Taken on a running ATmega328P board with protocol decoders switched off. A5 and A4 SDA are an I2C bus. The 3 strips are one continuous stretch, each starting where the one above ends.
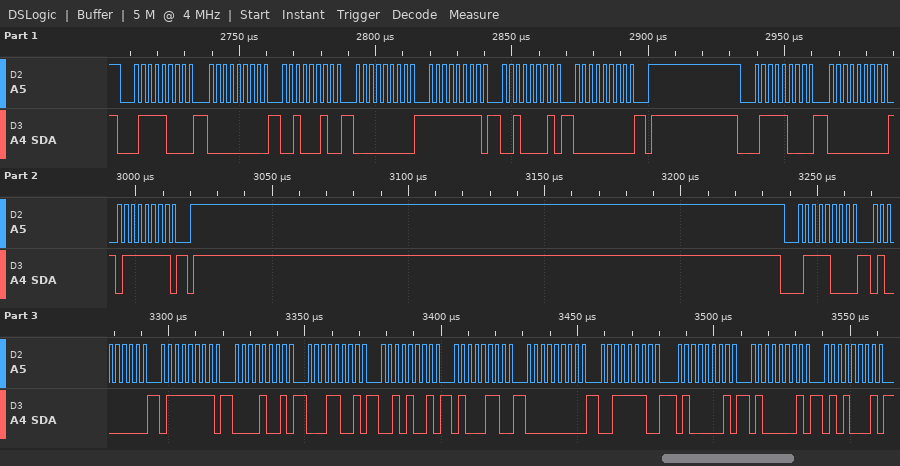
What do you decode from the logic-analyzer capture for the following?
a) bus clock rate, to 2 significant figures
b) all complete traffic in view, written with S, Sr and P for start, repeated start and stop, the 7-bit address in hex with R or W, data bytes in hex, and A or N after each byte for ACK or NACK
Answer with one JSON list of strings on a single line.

["400 kHz", "S 3CW A 00 A 22 A 00 A FF A 21 A 00 A P S 3CW A 00 A 7F A P S 3CW A 40 A 7F A 09 A 19 A 29 A 46 A 00 A 3E A 41 A 41 A 51 A"]
